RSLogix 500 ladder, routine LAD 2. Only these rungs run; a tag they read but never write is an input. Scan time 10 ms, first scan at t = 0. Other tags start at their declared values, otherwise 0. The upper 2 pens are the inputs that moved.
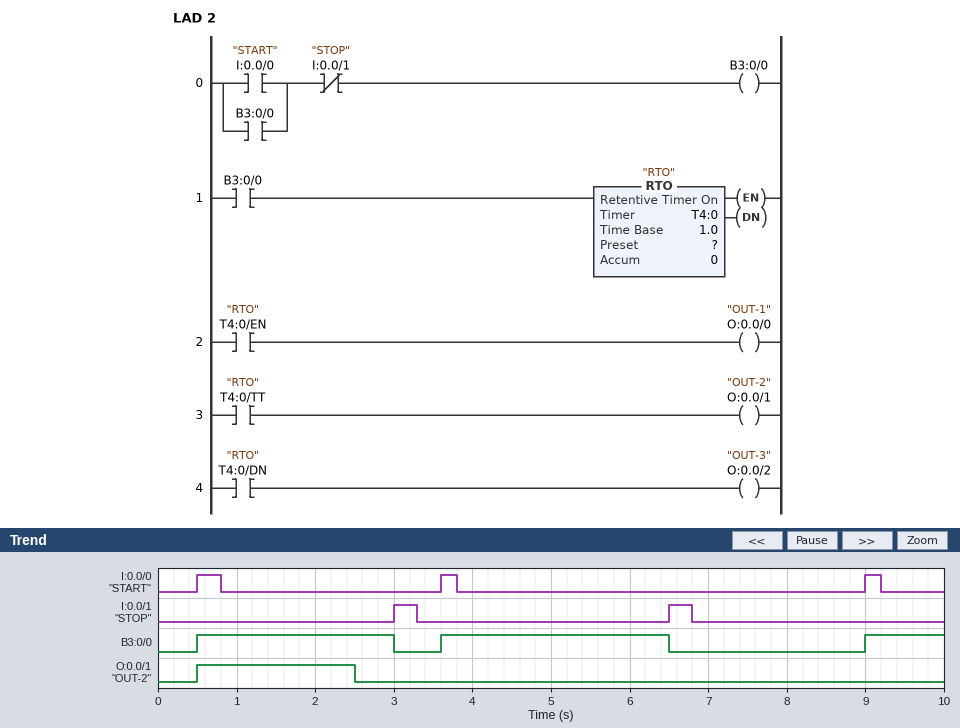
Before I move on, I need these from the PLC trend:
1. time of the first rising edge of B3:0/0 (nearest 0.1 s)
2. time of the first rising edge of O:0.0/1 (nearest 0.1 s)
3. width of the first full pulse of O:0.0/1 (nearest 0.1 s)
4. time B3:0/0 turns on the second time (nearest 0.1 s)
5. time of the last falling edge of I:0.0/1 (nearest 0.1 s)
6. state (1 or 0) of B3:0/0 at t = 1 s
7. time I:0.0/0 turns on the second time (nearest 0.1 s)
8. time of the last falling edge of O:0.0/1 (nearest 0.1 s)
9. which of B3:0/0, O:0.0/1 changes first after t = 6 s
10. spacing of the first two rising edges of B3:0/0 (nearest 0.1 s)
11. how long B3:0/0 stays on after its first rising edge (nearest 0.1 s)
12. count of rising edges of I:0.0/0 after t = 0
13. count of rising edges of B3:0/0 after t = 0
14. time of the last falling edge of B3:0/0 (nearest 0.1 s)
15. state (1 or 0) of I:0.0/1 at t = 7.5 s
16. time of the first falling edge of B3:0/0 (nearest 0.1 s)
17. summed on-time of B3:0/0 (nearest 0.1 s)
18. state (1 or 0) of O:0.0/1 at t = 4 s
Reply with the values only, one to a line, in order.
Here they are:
0.5 s
0.5 s
2.0 s
3.6 s
6.8 s
1
3.6 s
2.5 s
B3:0/0
3.1 s
2.5 s
3
3
6.5 s
0
3.0 s
6.4 s
0
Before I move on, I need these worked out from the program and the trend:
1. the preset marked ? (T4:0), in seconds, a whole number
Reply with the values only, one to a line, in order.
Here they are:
2 s
